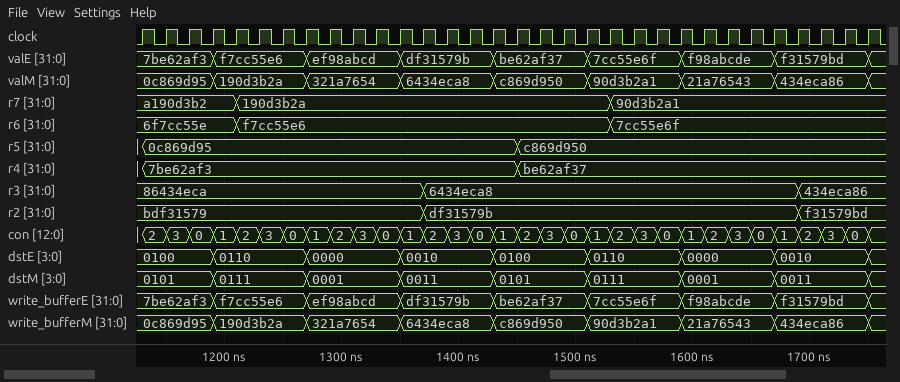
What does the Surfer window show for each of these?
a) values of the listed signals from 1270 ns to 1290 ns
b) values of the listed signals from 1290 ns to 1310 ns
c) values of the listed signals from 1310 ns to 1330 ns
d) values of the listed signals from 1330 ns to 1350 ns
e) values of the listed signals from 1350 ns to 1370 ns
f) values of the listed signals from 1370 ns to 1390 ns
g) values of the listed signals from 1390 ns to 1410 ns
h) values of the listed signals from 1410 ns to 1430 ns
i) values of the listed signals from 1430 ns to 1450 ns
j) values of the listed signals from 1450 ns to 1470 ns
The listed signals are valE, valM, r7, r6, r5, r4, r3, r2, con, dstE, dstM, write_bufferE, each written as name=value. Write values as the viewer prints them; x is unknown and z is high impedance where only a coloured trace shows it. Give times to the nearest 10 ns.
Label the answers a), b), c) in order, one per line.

a) valE=ef98abcd, valM=321a7654, r7=190d3b2a, r6=f7cc55e6, r5=0c869d95, r4=7be62af3, r3=86434eca, r2=bdf31579, con=1, dstE=0000, dstM=0001, write_bufferE=ef98abcd
b) valE=ef98abcd, valM=321a7654, r7=190d3b2a, r6=f7cc55e6, r5=0c869d95, r4=7be62af3, r3=86434eca, r2=bdf31579, con=2, dstE=0000, dstM=0001, write_bufferE=ef98abcd
c) valE=ef98abcd, valM=321a7654, r7=190d3b2a, r6=f7cc55e6, r5=0c869d95, r4=7be62af3, r3=86434eca, r2=bdf31579, con=3, dstE=0000, dstM=0001, write_bufferE=ef98abcd
d) valE=ef98abcd, valM=321a7654, r7=190d3b2a, r6=f7cc55e6, r5=0c869d95, r4=7be62af3, r3=86434eca, r2=bdf31579, con=0, dstE=0000, dstM=0001, write_bufferE=ef98abcd
e) valE=df31579b, valM=6434eca8, r7=190d3b2a, r6=f7cc55e6, r5=0c869d95, r4=7be62af3, r3=86434eca, r2=bdf31579, con=1, dstE=0010, dstM=0011, write_bufferE=df31579b
f) valE=df31579b, valM=6434eca8, r7=190d3b2a, r6=f7cc55e6, r5=0c869d95, r4=7be62af3, r3=6434eca8, r2=df31579b, con=2, dstE=0010, dstM=0011, write_bufferE=df31579b
g) valE=df31579b, valM=6434eca8, r7=190d3b2a, r6=f7cc55e6, r5=0c869d95, r4=7be62af3, r3=6434eca8, r2=df31579b, con=3, dstE=0010, dstM=0011, write_bufferE=df31579b
h) valE=df31579b, valM=6434eca8, r7=190d3b2a, r6=f7cc55e6, r5=0c869d95, r4=7be62af3, r3=6434eca8, r2=df31579b, con=0, dstE=0010, dstM=0011, write_bufferE=df31579b
i) valE=be62af37, valM=c869d950, r7=190d3b2a, r6=f7cc55e6, r5=0c869d95, r4=7be62af3, r3=6434eca8, r2=df31579b, con=1, dstE=0100, dstM=0101, write_bufferE=be62af37
j) valE=be62af37, valM=c869d950, r7=190d3b2a, r6=f7cc55e6, r5=c869d950, r4=be62af37, r3=6434eca8, r2=df31579b, con=2, dstE=0100, dstM=0101, write_bufferE=be62af37
